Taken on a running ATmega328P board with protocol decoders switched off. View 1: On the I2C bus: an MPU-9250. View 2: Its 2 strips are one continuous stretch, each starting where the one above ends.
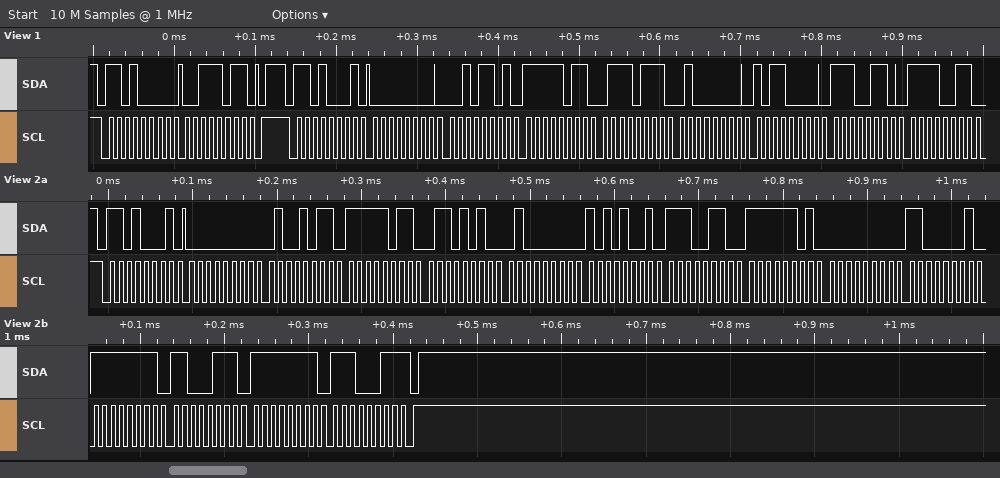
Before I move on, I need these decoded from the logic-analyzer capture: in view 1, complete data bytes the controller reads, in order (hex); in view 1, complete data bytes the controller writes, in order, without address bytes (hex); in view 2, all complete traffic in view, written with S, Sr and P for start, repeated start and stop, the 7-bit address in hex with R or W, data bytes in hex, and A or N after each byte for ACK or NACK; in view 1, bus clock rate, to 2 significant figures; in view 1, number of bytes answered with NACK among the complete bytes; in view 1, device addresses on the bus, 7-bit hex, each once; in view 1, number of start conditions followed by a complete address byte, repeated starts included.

00 2D FB 77 40 B0 E6 F3
3B
S 68R A 00 A 4B A FB A 6A A 40 A A9 A E6 A FD A 00 A C1 A FF A C7 A FF A E3 N P
100 kHz
0
0x68
2
